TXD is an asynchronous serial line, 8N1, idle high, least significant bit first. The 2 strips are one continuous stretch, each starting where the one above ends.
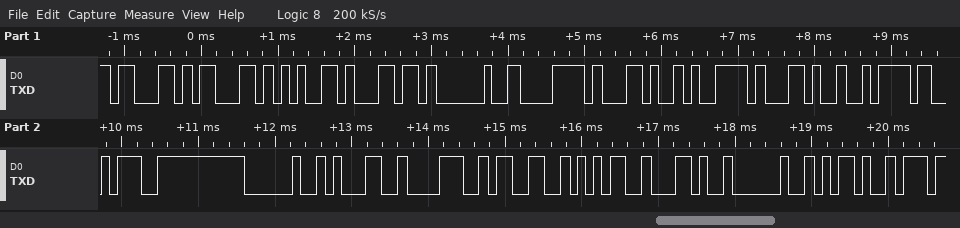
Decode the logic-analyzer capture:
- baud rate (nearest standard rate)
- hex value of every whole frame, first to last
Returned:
9600 baud
0x63 0x63 0x65 0x6C 0x20 0x78 0x2C 0x79 0x2C 0x7A 0x3A 0x20 0x31 0x38 0x33 0x35 0x2C 0x20 0x2D
